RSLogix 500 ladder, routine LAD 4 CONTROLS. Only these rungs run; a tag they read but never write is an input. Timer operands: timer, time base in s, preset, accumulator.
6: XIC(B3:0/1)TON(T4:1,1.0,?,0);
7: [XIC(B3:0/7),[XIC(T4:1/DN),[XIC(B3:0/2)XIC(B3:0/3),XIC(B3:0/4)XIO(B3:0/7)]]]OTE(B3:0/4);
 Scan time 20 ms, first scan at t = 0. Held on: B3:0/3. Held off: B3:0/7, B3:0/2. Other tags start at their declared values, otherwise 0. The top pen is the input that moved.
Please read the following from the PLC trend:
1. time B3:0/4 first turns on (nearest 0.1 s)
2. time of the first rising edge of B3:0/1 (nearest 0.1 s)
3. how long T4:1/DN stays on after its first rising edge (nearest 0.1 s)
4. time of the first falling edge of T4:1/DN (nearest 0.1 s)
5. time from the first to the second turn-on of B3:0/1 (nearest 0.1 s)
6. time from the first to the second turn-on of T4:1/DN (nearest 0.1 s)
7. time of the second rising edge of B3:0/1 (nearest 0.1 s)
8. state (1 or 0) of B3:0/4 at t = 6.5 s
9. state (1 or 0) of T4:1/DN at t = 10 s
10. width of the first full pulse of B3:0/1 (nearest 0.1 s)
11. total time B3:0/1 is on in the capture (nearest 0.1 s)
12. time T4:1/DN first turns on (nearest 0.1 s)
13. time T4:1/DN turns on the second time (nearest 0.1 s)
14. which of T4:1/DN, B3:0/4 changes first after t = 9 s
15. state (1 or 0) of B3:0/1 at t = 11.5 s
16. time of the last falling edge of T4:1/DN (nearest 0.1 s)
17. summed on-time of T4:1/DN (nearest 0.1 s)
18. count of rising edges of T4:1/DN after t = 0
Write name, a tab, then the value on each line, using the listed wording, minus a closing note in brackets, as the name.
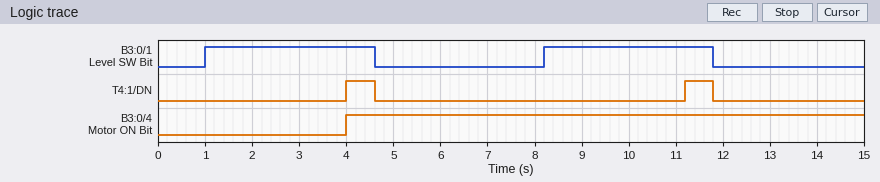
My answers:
time B3:0/4 first turns on	4.0 s
time of the first rising edge of B3:0/1	1.0 s
how long T4:1/DN stays on after its first rising edge	0.6 s
time of the first falling edge of T4:1/DN	4.6 s
time from the first to the second turn-on of B3:0/1	7.2 s
time from the first to the second turn-on of T4:1/DN	7.2 s
time of the second rising edge of B3:0/1	8.2 s
state (1 or 0) of B3:0/4 at t = 6.5 s	1
state (1 or 0) of T4:1/DN at t = 10 s	0
width of the first full pulse of B3:0/1	3.6 s
total time B3:0/1 is on in the capture	7.2 s
time T4:1/DN first turns on	4.0 s
time T4:1/DN turns on the second time	11.2 s
which of T4:1/DN, B3:0/4 changes first after t = 9 s	T4:1/DN
state (1 or 0) of B3:0/1 at t = 11.5 s	1
time of the last falling edge of T4:1/DN	11.8 s
summed on-time of T4:1/DN	1.2 s
count of rising edges of T4:1/DN after t = 0	2
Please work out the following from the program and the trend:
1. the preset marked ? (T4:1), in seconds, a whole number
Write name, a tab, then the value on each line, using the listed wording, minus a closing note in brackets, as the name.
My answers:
the preset marked ? (T4:1), in seconds, a whole number	3 s
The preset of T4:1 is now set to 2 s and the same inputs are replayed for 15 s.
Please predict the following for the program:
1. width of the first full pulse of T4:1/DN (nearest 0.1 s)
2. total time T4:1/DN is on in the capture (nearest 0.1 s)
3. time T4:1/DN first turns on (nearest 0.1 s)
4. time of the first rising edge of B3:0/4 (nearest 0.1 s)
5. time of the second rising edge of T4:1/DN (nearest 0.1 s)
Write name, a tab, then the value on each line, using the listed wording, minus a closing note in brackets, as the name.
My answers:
width of the first full pulse of T4:1/DN	1.6 s
total time T4:1/DN is on in the capture	3.2 s
time T4:1/DN first turns on	3.0 s
time of the first rising edge of B3:0/4	3.0 s
time of the second rising edge of T4:1/DN	10.2 s
